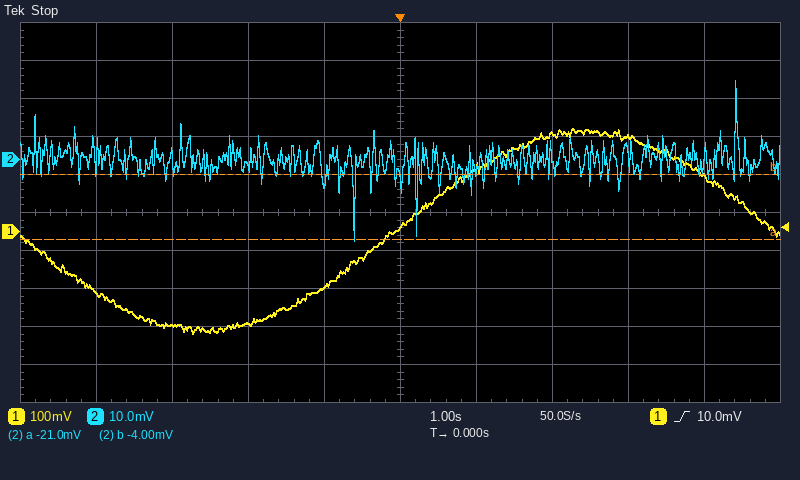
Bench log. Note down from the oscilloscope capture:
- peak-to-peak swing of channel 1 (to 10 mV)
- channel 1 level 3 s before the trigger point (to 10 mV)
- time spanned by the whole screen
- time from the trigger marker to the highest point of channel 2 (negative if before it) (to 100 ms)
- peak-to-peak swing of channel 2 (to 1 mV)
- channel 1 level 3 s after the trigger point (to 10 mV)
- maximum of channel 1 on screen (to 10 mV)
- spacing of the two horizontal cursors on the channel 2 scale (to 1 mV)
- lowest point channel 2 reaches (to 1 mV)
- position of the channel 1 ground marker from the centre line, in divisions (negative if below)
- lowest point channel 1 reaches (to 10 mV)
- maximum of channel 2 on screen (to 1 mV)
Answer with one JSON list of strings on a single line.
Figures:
["540 mV", "-250 mV", "10 s", "+4.4 s", "42 mV", "250 mV", "270 mV", "17 mV", "-21 mV", "-0.5 div", "-270 mV", "21 mV"]
